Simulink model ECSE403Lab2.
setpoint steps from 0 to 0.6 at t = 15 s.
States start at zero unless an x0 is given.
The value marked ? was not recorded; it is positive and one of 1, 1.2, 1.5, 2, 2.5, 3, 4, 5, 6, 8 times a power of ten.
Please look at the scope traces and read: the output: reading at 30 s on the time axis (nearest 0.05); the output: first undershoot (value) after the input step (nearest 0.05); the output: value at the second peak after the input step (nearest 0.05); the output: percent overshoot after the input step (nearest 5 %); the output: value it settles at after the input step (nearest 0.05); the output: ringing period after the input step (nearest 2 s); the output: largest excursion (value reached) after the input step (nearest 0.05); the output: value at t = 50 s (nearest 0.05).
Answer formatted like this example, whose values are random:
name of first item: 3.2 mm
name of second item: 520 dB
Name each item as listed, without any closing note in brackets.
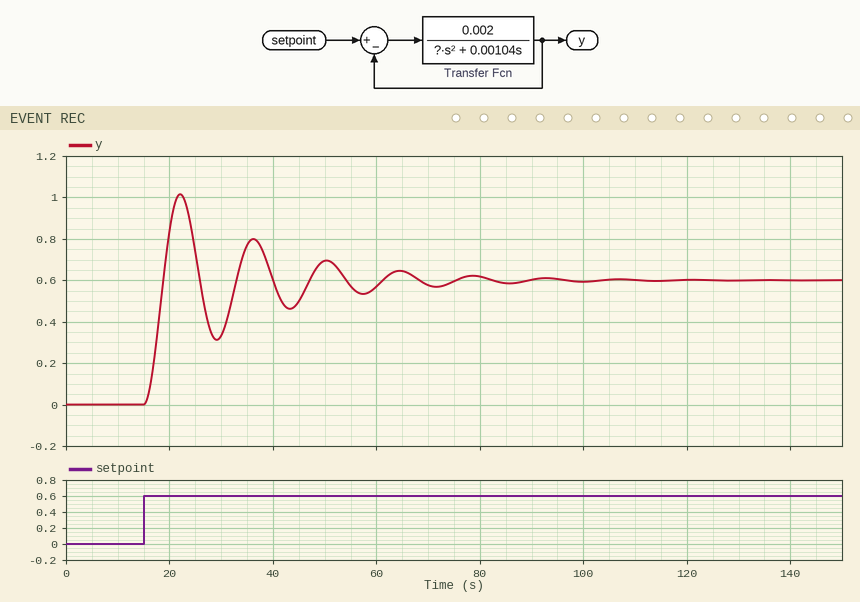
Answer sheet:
the output: reading at 30 s on the time axis: 0.35
the output: first undershoot (value) after the input step: 0.30
the output: value at the second peak after the input step: 0.80
the output: percent overshoot after the input step: 70 %
the output: value it settles at after the input step: 0.60
the output: ringing period after the input step: 14 s
the output: largest excursion (value reached) after the input step: 1.00
the output: value at t = 50 s: 0.70
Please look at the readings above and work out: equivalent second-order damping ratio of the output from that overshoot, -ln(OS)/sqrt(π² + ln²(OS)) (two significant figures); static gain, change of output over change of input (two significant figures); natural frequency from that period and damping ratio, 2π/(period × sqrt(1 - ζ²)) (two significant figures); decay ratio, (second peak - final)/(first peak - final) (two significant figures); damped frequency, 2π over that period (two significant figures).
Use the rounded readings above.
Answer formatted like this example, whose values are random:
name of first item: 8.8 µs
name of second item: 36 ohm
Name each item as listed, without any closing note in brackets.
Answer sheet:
equivalent second-order damping ratio of the output from that overshoot, -ln(OS)/sqrt(π² + ln²(OS)): 0.11
static gain, change of output over change of input: 1.0
natural frequency from that period and damping ratio, 2π/(period × sqrt(1 - ζ²)): 0.45 rad/s
decay ratio, (second peak - final)/(first peak - final): 0.50
damped frequency, 2π over that period: 0.45 rad/s
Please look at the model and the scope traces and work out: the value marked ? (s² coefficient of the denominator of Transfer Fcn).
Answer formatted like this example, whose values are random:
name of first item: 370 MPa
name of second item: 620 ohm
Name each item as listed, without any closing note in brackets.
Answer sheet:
the value marked ?: 0.01
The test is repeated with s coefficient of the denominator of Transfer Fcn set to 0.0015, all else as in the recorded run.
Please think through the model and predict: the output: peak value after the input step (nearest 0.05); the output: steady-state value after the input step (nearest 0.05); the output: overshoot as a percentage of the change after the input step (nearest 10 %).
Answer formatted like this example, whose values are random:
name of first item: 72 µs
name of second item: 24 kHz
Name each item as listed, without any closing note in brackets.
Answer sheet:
the output: peak value after the input step: 0.95
the output: steady-state value after the input step: 0.60
the output: overshoot as a percentage of the change after the input step: 60 %
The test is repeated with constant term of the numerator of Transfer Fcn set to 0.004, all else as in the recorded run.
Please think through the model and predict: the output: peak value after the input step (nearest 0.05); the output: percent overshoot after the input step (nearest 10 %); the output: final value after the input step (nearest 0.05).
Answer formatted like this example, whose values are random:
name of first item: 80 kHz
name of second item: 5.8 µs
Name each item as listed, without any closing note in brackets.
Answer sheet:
the output: peak value after the input step: 1.05
the output: percent overshoot after the input step: 80 %
the output: final value after the input step: 0.60
